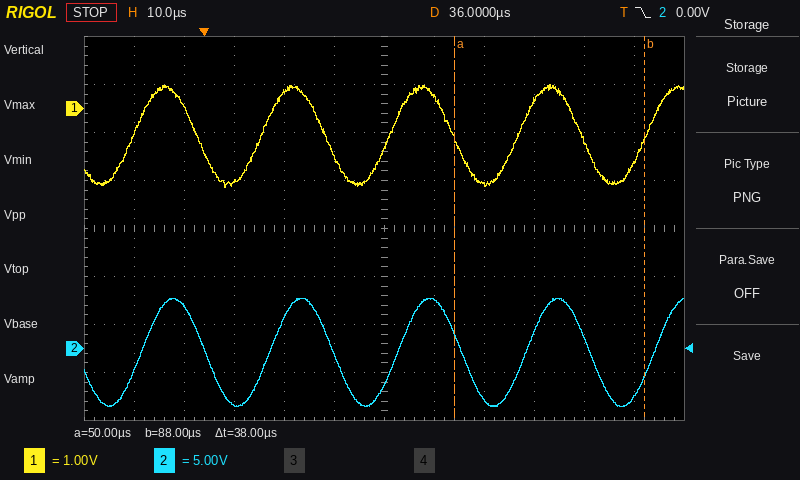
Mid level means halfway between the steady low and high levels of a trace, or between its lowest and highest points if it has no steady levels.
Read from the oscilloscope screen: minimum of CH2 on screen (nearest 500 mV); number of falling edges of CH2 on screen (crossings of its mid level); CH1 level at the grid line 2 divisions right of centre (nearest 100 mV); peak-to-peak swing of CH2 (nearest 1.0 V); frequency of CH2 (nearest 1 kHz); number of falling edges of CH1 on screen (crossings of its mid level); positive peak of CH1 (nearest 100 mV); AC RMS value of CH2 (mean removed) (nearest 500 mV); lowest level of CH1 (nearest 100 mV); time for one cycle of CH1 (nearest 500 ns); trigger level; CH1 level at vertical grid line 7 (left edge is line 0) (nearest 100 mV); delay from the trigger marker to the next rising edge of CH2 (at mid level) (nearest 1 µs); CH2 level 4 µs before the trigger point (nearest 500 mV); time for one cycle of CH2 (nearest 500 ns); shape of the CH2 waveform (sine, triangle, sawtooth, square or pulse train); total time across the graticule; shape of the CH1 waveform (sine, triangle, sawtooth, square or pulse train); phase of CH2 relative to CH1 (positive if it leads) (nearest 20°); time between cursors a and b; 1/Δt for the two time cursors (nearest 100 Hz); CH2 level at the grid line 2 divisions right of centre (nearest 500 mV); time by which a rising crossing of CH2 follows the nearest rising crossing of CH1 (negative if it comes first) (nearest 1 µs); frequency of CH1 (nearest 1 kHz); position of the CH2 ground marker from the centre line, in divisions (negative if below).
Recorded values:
-6.0 V
4
-1.6 V
11.0 V
39 kHz
4
500 mV
4.0 V
-1.6 V
25.5 µs
0.00 V
200 mV
13 µs
4.5 V
25.5 µs
sine
120 µs
sine
-20°
38 µs
26.3 kHz
-5.5 V
+2 µs
39 kHz
-2.5 div
